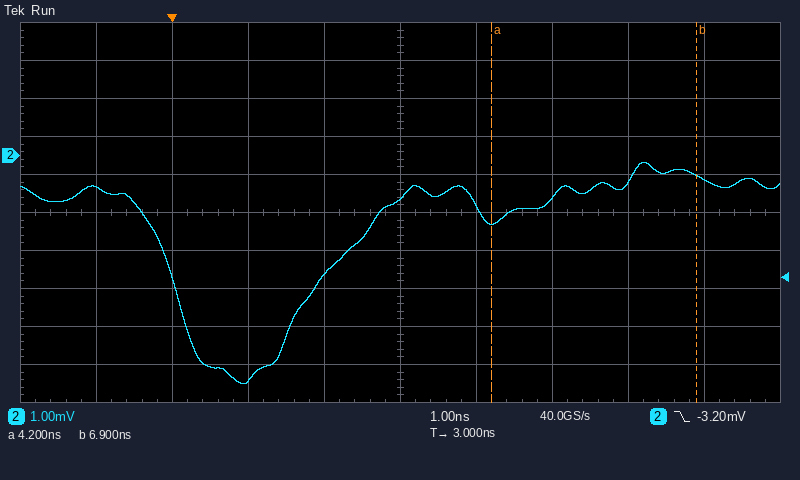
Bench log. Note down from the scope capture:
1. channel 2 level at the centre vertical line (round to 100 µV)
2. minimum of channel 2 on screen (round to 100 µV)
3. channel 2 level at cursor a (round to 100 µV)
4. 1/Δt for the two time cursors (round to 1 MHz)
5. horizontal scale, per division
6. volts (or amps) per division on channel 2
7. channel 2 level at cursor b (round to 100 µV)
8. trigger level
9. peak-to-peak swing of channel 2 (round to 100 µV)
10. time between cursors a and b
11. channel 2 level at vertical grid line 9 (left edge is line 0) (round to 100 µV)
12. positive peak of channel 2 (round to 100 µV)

-1.1 mV
-6.0 mV
-1.8 mV
370 MHz
1 ns
1 mV
-500 µV
-3.20 mV
5.8 mV
2.7 ns
-600 µV
-200 µV
